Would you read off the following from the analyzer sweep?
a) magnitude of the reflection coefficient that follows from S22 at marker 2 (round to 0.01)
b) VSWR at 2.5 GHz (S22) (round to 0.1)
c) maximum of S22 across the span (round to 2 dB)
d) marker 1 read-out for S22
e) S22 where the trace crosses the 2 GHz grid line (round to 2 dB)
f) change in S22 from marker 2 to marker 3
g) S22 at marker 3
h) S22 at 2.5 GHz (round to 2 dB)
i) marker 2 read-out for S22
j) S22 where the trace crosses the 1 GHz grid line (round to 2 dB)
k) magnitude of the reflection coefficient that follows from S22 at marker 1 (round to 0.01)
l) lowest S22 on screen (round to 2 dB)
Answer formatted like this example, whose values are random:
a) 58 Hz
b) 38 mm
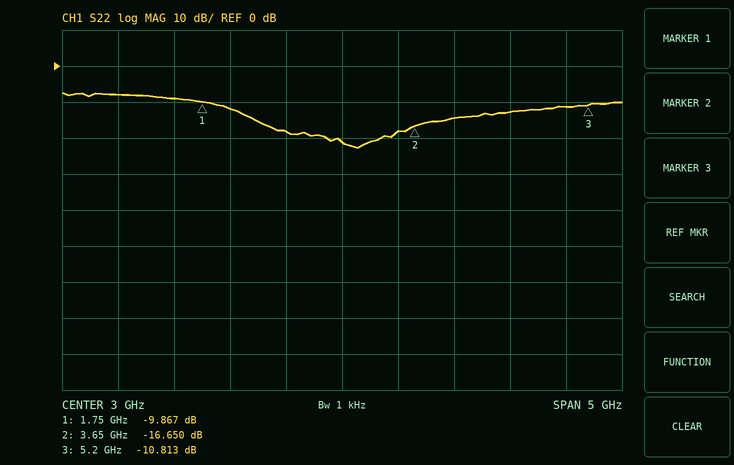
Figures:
a) 0.15
b) 1.3
c) -8 dB
d) -9.867 dB
e) -12 dB
f) 5.837 dB
g) -10.813 dB
h) -18 dB
i) -16.650 dB
j) -8 dB
k) 0.32
l) -22 dB
